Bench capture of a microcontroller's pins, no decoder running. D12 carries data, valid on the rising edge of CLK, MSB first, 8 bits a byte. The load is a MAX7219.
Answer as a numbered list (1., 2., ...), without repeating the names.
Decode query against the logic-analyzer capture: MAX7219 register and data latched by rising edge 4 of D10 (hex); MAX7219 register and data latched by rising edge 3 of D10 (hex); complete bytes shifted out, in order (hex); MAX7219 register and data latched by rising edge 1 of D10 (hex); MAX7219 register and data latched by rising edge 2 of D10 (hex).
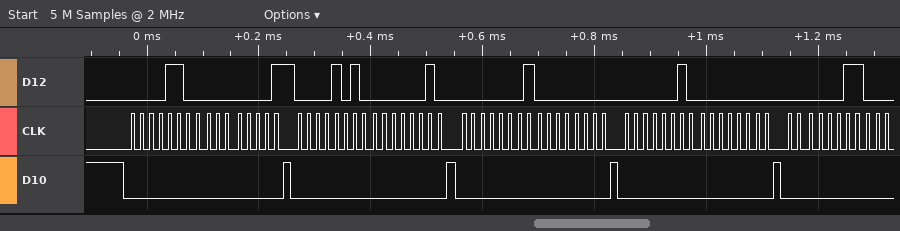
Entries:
1. register 0x2, data 0x00
2. register 0x1, data 0x00
3. 0C 01 0A 02 01 00 02 00 03
4. register 0xC, data 0x01
5. register 0xA, data 0x02
